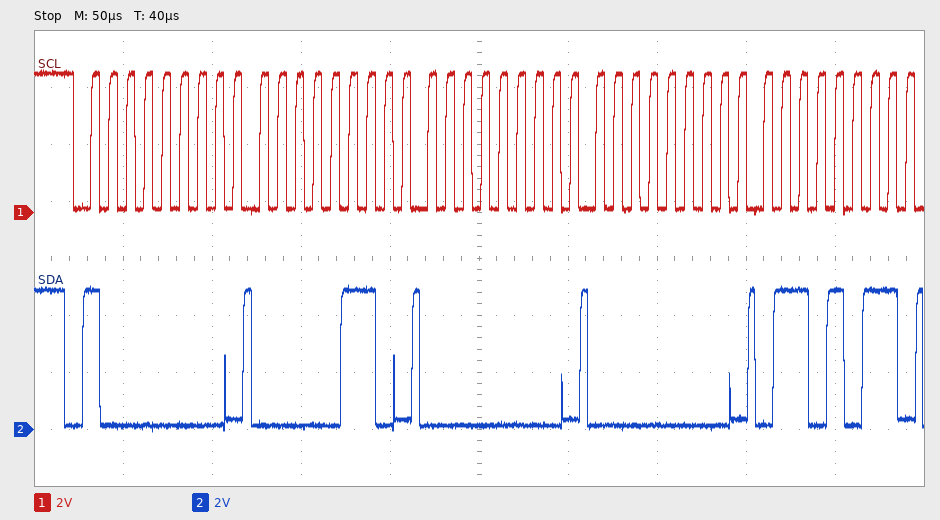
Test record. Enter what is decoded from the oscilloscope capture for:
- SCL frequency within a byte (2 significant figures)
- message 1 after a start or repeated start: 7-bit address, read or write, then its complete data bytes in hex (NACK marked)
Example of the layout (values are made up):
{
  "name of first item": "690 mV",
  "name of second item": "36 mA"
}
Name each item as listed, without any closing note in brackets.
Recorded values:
{
  "SCL frequency within a byte": "100 kHz",
  "message 1 after a start or repeated start: 7-bit address, read or write, then its complete data bytes in hex": "0x40 write: 06 00 00 6B"
}
